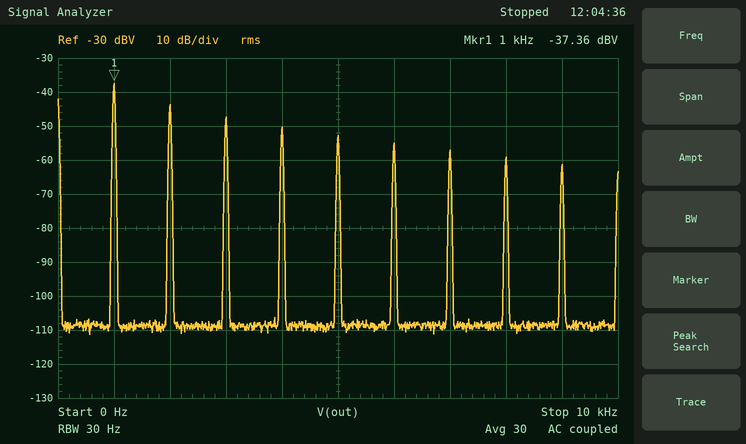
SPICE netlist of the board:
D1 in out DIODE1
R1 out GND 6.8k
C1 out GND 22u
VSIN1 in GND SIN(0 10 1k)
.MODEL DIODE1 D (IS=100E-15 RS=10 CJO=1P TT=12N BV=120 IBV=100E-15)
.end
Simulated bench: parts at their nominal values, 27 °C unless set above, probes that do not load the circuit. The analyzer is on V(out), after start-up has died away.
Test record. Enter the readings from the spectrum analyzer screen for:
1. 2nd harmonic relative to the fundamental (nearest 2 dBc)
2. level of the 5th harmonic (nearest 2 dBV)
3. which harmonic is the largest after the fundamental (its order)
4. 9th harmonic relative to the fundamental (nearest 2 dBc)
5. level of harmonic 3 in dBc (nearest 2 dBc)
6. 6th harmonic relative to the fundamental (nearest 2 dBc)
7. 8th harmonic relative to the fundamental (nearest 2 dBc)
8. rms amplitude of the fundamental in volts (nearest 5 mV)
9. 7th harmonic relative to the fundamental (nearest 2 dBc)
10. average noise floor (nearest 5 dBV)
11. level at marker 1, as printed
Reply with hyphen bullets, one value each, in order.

- -6 dBc
- -52 dBV
- 2
- -24 dBc
- -10 dBc
- -18 dBc
- -22 dBc
- 15 mV
- -20 dBc
- -110 dBV
- -37.36 dBV
